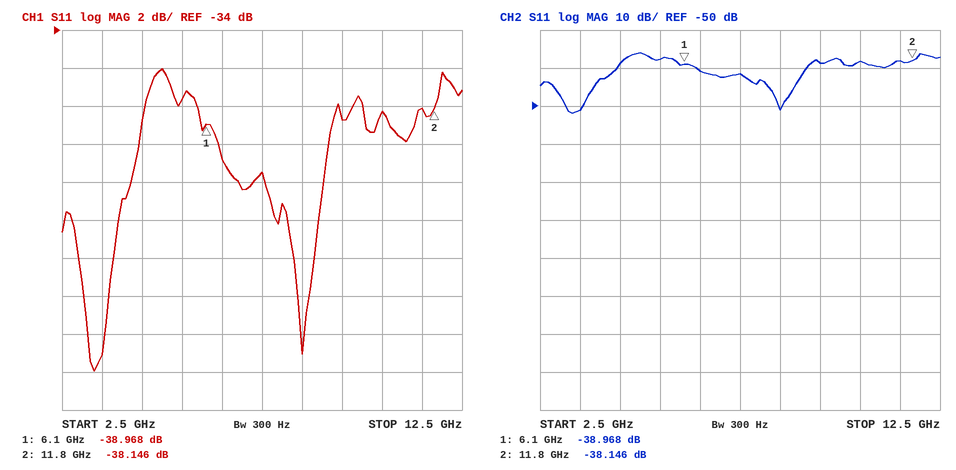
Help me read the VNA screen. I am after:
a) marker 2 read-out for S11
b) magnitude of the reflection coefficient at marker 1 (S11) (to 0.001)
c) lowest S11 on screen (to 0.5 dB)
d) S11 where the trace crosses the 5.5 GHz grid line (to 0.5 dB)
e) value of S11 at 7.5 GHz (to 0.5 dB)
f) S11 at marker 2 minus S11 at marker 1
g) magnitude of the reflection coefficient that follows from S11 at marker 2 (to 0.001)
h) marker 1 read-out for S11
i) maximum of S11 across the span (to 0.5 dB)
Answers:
-38.146 dB
0.011
-52.0 dB
-37.5 dB
-41.5 dB
0.822 dB
0.012
-38.968 dB
-36.0 dB
